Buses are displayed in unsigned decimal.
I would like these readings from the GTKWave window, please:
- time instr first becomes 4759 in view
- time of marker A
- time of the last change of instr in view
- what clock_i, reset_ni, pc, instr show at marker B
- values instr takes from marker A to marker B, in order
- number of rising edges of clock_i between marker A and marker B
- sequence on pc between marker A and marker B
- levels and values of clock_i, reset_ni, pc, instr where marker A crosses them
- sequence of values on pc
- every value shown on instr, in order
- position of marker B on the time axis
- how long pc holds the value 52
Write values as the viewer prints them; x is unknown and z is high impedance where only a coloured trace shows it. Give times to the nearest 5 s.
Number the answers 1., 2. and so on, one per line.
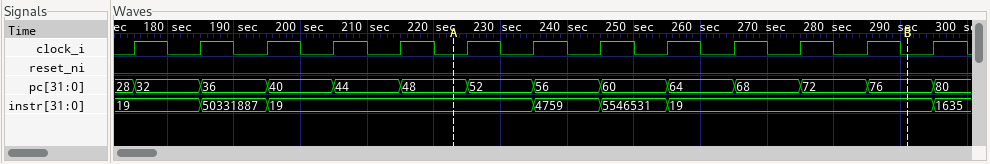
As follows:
1. 235 s
2. 225 s
3. 295 s
4. clock_i=0, reset_ni=0, pc=76, instr=19
5. 19, 4759, 5546531, 19
6. 7
7. 48, 52, 56, 60, 64, 68, 72, 76
8. clock_i=0, reset_ni=0, pc=48, instr=19
9. 28, 32, 36, 40, 44, 48, 52, 56, 60, 64, 68, 72, 76, 80
10. 19, 50331887, 19, 4759, 5546531, 19, 1635
11. 290 s
12. 10 s
